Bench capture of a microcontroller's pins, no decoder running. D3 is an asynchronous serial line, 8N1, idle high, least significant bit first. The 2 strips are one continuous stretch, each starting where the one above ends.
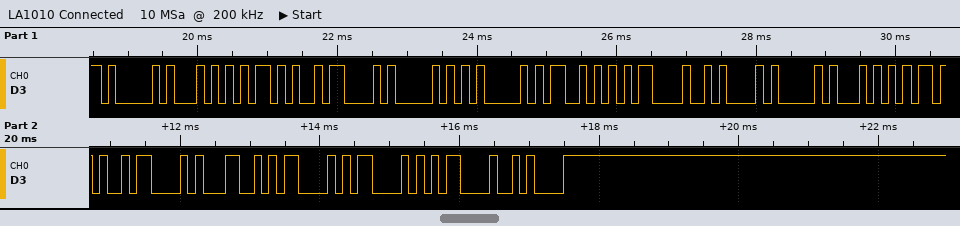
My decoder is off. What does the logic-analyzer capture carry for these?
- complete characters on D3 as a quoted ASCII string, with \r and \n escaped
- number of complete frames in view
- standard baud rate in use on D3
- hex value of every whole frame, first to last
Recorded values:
"AT+CPAS\r\nAT+CLCC\r\n"
18
9600 baud
0x41 0x54 0x2B 0x43 0x50 0x41 0x53 0x0D 0x0A 0x41 0x54 0x2B 0x43 0x4C 0x43 0x43 0x0D 0x0A
